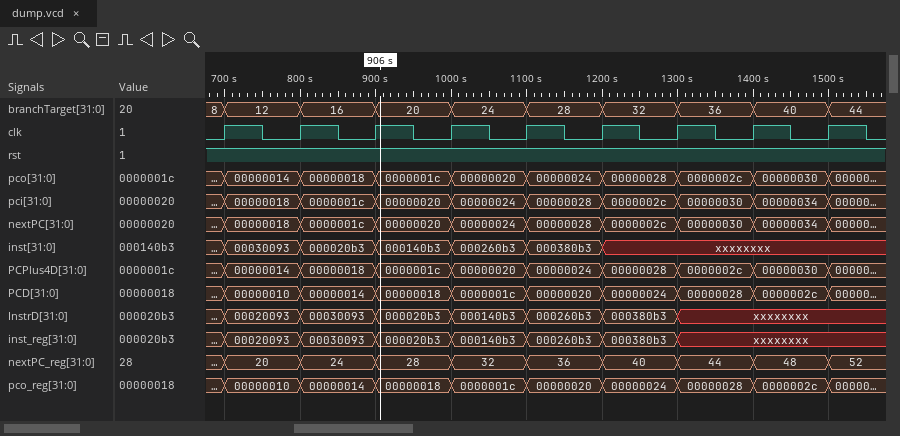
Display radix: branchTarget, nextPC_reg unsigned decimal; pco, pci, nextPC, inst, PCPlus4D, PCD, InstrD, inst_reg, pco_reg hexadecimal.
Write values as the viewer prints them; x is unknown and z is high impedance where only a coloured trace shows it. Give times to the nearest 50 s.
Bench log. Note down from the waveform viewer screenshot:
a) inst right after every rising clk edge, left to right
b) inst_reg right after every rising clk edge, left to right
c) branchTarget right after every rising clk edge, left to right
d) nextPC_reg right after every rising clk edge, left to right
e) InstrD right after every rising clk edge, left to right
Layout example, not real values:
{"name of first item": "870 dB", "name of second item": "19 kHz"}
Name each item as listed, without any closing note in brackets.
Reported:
{"inst right after every rising clk edge, left to right": "00030093, 000020b3, 000140b3, 000260b3, 000380b3, xxxxxxxx, xxxxxxxx, xxxxxxxx, xxxxxxxx", "inst_reg right after every rising clk edge, left to right": "00020093, 00030093, 000020b3, 000140b3, 000260b3, 000380b3, xxxxxxxx, xxxxxxxx, xxxxxxxx", "branchTarget right after every rising clk edge, left to right": "12, 16, 20, 24, 28, 32, 36, 40, 44", "nextPC_reg right after every rising clk edge, left to right": "20, 24, 28, 32, 36, 40, 44, 48, 52", "InstrD right after every rising clk edge, left to right": "00020093, 00030093, 000020b3, 000140b3, 000260b3, 000380b3, xxxxxxxx, xxxxxxxx, xxxxxxxx"}
